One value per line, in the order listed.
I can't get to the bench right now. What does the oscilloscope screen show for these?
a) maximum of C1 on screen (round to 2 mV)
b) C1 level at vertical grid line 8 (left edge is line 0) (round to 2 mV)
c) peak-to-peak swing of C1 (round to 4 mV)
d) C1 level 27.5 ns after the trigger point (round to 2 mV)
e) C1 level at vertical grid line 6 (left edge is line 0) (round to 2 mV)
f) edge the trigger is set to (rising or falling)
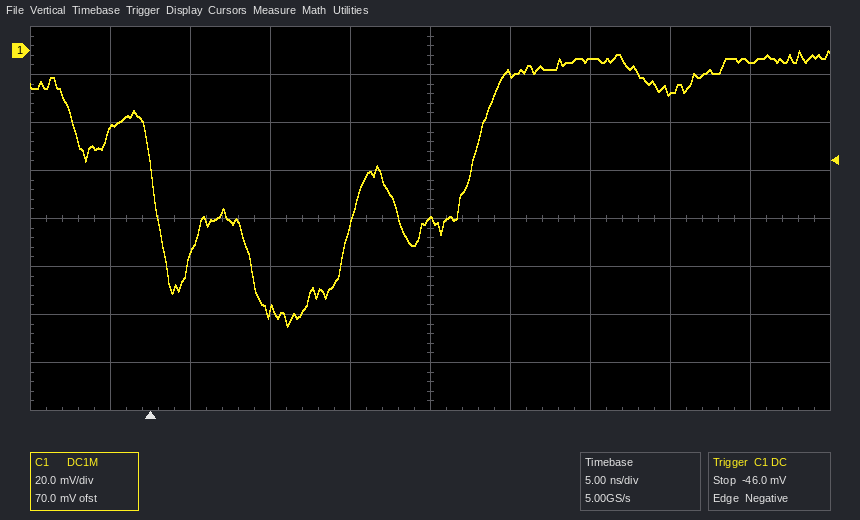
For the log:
0 mV
-18 mV
116 mV
-4 mV
-10 mV
falling
